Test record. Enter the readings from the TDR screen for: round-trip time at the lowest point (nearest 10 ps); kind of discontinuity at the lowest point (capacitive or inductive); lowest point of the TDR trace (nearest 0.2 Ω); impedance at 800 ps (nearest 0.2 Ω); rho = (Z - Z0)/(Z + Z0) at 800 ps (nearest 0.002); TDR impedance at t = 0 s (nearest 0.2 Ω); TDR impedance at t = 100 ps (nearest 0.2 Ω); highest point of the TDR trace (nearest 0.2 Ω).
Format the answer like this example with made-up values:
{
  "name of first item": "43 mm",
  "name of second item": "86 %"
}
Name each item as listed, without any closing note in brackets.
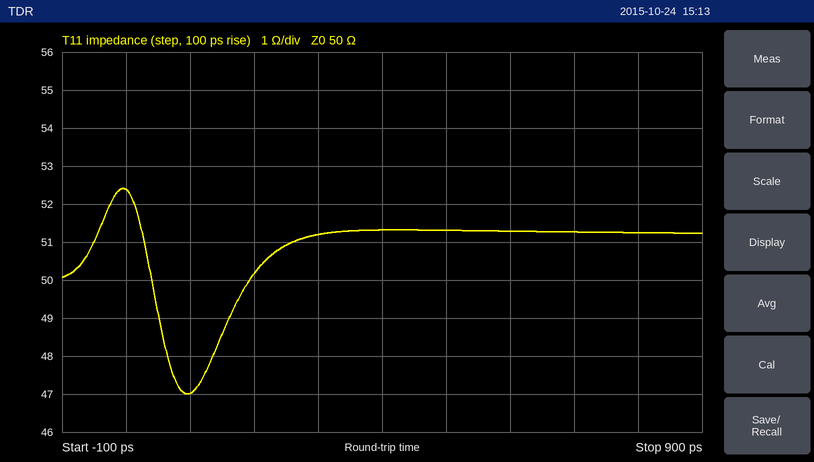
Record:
{
  "round-trip time at the lowest point": "100 ps",
  "kind of discontinuity at the lowest point": "capacitive",
  "lowest point of the TDR trace": "47.0 Ω",
  "impedance at 800 ps": "51.2 Ω",
  "rho = (Z - Z0)/(Z + Z0) at 800 ps": "+0.012",
  "TDR impedance at t = 0 s": "52.4 Ω",
  "TDR impedance at t = 100 ps": "47.0 Ω",
  "highest point of the TDR trace": "52.4 Ω"
}
